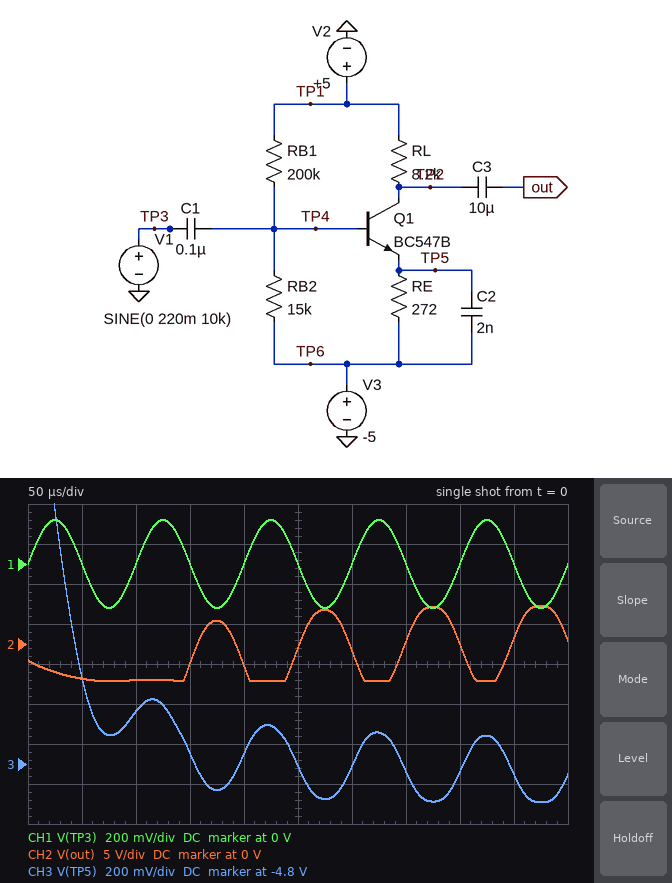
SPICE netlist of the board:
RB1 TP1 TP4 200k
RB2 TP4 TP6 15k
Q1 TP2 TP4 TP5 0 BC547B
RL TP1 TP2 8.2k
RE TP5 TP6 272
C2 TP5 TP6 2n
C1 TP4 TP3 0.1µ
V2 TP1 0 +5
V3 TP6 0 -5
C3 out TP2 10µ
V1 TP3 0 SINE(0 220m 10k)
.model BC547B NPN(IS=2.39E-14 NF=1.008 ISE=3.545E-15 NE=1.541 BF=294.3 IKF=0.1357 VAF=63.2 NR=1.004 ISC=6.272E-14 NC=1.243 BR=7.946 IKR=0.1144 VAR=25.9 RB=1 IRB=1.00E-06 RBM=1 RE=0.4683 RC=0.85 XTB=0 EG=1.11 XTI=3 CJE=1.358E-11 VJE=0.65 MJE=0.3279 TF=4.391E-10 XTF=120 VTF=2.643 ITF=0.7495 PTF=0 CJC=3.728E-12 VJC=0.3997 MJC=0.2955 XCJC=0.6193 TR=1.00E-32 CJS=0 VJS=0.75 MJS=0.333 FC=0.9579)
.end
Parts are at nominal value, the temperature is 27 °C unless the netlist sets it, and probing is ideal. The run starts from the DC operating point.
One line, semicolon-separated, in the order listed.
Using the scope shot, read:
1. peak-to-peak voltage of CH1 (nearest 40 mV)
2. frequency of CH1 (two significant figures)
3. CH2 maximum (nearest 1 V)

440 mV; 10 kHz; 5 V
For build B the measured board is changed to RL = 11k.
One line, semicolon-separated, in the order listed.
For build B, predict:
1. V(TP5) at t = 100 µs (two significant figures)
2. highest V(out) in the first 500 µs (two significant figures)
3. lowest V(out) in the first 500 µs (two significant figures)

-4.6 V; 5.0 V; -4.7 V
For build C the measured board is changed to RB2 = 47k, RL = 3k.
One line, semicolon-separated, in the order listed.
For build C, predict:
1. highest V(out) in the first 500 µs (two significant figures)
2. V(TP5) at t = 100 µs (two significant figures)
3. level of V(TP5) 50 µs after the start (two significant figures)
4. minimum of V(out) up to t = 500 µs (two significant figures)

100 mV; -4.0 V; -3.9 V; -4.1 V
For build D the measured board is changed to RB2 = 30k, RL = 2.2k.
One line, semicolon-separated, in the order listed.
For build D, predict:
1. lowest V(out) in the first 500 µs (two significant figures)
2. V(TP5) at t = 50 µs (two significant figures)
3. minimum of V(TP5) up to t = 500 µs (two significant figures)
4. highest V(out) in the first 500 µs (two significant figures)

-3.8 V; -3.7 V; -4.3 V; -320 mV
